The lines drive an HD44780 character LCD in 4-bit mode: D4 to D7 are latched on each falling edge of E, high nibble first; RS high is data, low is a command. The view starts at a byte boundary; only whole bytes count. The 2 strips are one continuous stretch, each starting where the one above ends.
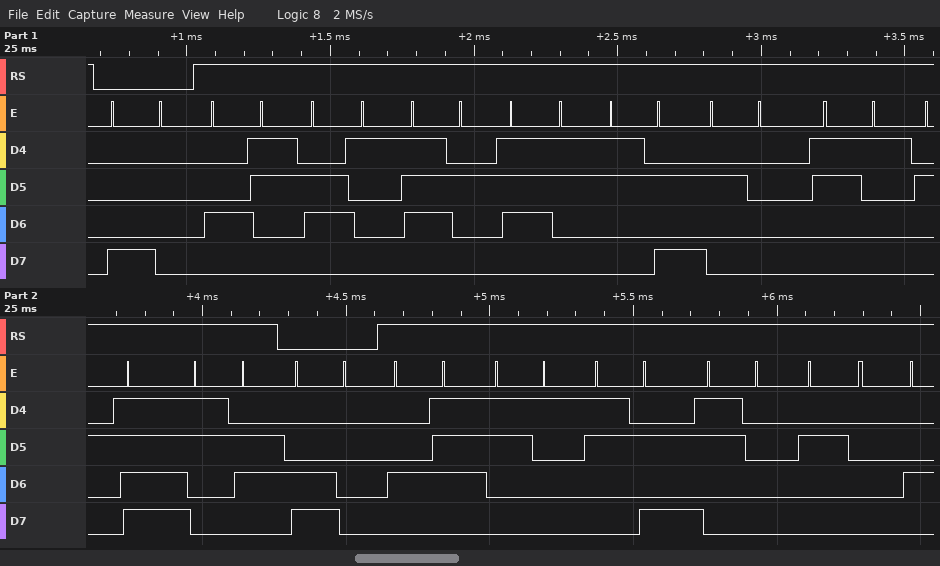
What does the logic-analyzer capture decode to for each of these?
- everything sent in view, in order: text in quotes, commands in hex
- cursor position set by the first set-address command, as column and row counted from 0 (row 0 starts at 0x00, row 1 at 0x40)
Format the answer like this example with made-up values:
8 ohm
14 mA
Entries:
0x80 "Cars: 1/6" 0xC0 "G1:0 "
column 0, row 0
